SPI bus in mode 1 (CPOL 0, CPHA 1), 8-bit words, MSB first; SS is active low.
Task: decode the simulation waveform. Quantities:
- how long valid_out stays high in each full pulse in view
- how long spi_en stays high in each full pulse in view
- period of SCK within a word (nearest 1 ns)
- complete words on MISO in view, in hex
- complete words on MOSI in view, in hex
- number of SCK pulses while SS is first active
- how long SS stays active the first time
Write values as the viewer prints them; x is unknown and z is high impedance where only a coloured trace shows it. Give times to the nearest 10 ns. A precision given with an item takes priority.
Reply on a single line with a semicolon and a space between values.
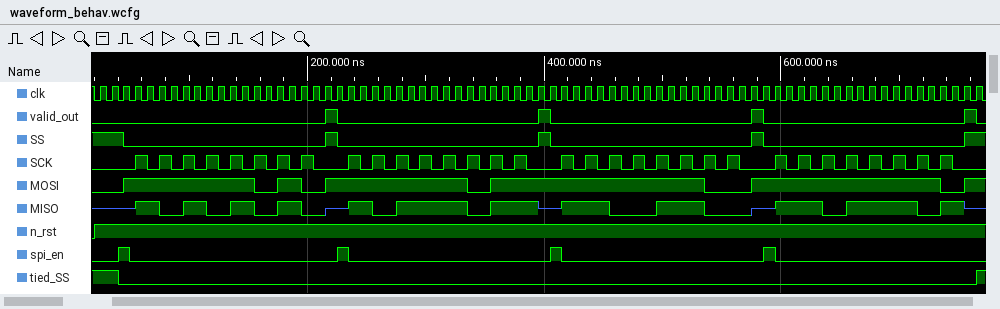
10 ns, 10 ns, 10 ns, 10 ns; 10 ns, 10 ns, 10 ns, 10 ns; 20 ns; AA, BB, CC, DD; FA, FB, FC, FE; 8; 170 ns
